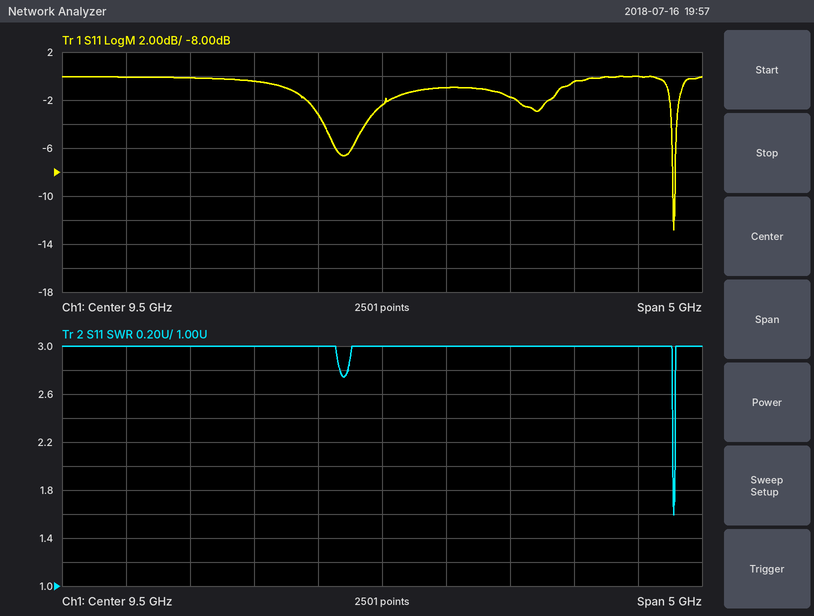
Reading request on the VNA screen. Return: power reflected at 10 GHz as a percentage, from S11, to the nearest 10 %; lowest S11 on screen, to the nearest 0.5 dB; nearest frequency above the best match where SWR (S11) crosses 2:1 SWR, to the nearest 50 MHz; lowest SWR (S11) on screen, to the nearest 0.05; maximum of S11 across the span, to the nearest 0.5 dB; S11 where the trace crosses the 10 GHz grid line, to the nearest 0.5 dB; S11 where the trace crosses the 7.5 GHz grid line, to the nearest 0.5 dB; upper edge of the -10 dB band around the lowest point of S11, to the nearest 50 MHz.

80 %
-13.0 dB
11.80 GHz
1.60
0.0 dB
-1.0 dB
0.0 dB
11.80 GHz
